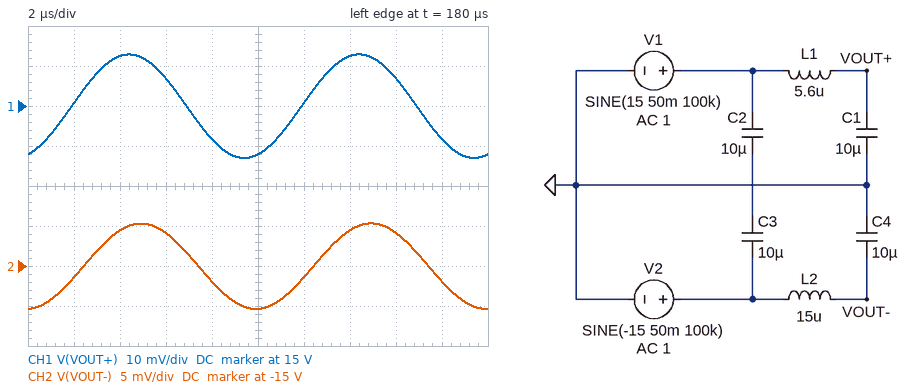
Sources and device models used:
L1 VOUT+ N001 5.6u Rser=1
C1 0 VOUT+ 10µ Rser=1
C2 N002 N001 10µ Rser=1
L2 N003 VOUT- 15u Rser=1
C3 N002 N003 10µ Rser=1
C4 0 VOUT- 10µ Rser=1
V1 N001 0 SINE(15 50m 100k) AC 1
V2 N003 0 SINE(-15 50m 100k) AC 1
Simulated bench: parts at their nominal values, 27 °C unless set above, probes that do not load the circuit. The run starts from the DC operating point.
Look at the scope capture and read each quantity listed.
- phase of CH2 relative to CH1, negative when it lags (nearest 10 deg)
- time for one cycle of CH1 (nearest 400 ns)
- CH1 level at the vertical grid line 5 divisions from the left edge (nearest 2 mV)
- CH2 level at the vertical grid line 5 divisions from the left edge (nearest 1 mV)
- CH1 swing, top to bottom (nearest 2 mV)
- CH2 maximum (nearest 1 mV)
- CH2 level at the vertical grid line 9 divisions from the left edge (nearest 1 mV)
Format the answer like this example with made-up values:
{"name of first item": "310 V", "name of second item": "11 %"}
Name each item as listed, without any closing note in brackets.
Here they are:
{"phase of CH2 relative to CH1, negative when it lags": "-20 deg", "time for one cycle of CH1": "10.0 µs", "CH1 level at the vertical grid line 5 divisions from the left edge": "14.988 V", "CH2 level at the vertical grid line 5 divisions from the left edge": "-15.005 V", "CH1 swing, top to bottom": "26 mV", "CH2 maximum": "-14.995 V", "CH2 level at the vertical grid line 9 divisions from the left edge": "-15.002 V"}
